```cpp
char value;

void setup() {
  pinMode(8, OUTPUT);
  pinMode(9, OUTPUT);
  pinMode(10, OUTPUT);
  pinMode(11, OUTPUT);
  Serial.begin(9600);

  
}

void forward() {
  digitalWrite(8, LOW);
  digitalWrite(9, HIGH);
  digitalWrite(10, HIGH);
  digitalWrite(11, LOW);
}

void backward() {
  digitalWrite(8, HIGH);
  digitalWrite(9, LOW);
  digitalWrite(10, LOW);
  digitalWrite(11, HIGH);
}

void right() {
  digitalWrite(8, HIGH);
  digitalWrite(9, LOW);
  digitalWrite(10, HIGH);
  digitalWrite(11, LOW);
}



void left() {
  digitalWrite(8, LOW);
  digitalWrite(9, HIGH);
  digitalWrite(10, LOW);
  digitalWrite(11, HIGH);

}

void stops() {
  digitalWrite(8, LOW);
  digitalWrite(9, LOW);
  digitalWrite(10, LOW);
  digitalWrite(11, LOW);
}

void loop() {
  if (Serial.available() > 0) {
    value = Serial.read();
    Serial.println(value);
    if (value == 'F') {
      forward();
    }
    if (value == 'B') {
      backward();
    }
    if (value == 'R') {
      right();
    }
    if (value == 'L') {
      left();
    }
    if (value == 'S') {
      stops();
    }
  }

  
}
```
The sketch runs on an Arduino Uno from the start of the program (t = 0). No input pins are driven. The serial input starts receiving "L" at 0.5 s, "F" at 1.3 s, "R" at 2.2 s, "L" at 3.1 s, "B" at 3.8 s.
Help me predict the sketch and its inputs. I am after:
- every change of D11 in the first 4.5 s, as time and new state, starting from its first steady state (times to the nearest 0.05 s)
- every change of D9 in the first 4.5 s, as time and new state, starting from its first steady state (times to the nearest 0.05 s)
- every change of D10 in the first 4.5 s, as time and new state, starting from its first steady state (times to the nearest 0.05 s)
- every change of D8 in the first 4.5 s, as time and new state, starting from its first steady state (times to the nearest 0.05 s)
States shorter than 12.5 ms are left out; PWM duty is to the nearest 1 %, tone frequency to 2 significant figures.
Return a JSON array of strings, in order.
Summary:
["0 s low; 0.5 s high; 1.3 s low; 3.1 s high", "0 s low; 0.5 s high; 2.2 s low; 3.1 s high; 3.8 s low", "0 s low; 1.3 s high; 3.1 s low", "0 s low; 2.2 s high; 3.1 s low; 3.8 s high"]
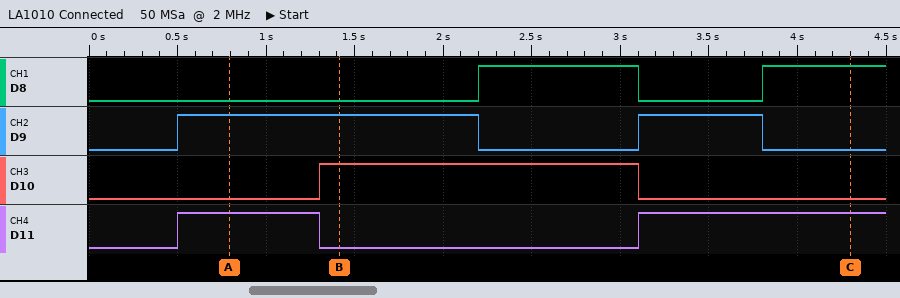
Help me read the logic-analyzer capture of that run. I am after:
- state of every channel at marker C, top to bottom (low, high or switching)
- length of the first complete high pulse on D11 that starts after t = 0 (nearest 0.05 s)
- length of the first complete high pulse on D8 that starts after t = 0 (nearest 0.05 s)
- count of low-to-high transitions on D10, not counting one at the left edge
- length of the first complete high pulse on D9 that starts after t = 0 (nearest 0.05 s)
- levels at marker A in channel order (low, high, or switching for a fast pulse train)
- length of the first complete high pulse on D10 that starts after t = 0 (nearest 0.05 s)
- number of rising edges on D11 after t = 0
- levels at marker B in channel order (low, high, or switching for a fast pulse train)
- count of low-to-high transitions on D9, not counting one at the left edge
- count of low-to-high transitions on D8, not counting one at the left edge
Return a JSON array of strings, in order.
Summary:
["D8 high, D9 low, D10 low, D11 high", "0.80 s", "0.90 s", "1", "1.70 s", "D8 low, D9 high, D10 low, D11 high", "1.80 s", "2", "D8 low, D9 high, D10 high, D11 low", "2", "2"]
